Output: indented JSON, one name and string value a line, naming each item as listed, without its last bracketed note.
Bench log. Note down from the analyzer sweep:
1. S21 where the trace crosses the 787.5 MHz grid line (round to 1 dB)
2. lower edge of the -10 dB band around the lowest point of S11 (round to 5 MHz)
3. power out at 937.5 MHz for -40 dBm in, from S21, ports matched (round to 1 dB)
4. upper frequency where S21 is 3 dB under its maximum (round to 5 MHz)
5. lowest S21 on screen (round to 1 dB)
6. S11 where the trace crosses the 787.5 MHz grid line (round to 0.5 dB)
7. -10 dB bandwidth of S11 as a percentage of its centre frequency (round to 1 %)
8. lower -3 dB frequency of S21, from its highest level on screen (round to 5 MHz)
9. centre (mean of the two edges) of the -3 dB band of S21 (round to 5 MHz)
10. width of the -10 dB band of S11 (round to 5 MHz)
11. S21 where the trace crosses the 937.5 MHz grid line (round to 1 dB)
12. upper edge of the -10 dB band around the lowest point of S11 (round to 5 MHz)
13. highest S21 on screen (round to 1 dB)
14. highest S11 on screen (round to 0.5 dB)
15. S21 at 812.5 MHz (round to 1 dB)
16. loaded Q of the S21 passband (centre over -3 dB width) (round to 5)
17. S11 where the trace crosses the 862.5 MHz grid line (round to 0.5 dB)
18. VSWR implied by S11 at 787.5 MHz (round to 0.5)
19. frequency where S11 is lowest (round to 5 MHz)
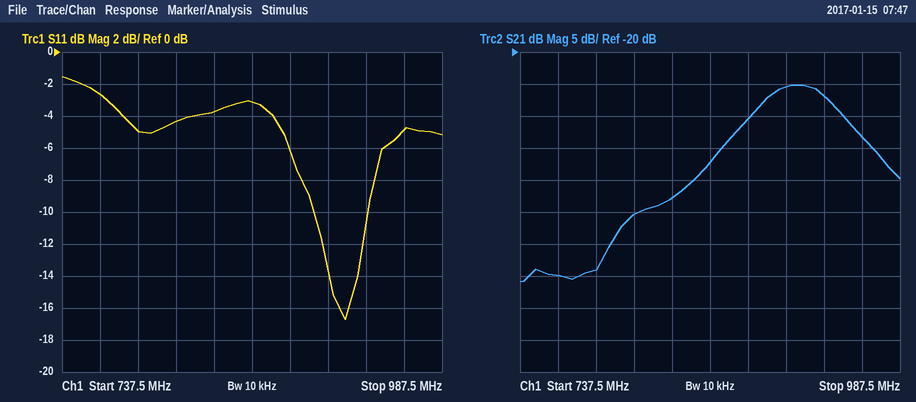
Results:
{
  "S21 where the trace crosses the 787.5 MHz grid line": "-54 dB",
  "lower edge of the -10 dB band around the lowest point of S11": "905 MHz",
  "power out at 937.5 MHz for -40 dBm in, from S21, ports matched": "-67 dBm",
  "upper frequency where S21 is 3 dB under its maximum": "945 MHz",
  "lowest S21 on screen": "-56 dB",
  "S11 where the trace crosses the 787.5 MHz grid line": "-5.0 dB",
  "-10 dB bandwidth of S11 as a percentage of its centre frequency": "4 %",
  "lower -3 dB frequency of S21, from its highest level on screen": "895 MHz",
  "centre (mean of the two edges) of the -3 dB band of S21": "920 MHz",
  "width of the -10 dB band of S11": "35 MHz",
  "S21 where the trace crosses the 937.5 MHz grid line": "-27 dB",
  "upper edge of the -10 dB band around the lowest point of S11": "940 MHz",
  "highest S21 on screen": "-25 dB",
  "highest S11 on screen": "-1.5 dB",
  "S21 at 812.5 MHz": "-45 dB",
  "loaded Q of the S21 passband (centre over -3 dB width)": "20",
  "S11 where the trace crosses the 862.5 MHz grid line": "-3.0 dB",
  "VSWR implied by S11 at 787.5 MHz": "3.5",
  "frequency where S11 is lowest": "925 MHz"
}
